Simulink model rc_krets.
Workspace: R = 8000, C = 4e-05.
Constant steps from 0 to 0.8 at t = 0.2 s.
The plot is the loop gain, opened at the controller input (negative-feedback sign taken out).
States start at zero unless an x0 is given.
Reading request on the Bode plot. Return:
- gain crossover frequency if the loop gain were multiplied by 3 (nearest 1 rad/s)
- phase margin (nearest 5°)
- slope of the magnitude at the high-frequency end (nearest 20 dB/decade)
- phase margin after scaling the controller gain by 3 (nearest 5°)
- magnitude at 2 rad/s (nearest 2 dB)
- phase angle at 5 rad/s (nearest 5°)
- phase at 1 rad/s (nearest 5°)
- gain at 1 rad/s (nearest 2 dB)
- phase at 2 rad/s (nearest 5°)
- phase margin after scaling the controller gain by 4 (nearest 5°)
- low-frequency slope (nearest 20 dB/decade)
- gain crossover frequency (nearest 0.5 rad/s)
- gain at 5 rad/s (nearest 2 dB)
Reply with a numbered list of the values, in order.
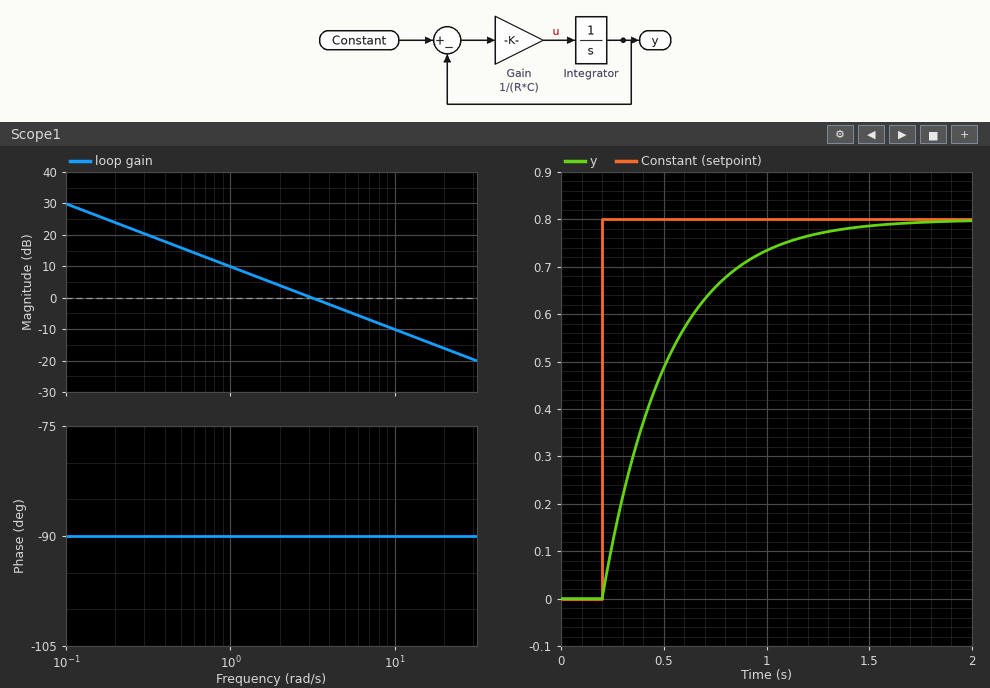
1. 9 rad/s
2. 90°
3. -20 dB/decade
4. 90°
5. 4 dB
6. -90°
7. -90°
8. 10 dB
9. -90°
10. 90°
11. -20 dB/decade
12. 3.0 rad/s
13. -4 dB
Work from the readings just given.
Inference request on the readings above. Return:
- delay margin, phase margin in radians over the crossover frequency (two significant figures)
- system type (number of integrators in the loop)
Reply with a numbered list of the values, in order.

1. 0.52 s
2. 1
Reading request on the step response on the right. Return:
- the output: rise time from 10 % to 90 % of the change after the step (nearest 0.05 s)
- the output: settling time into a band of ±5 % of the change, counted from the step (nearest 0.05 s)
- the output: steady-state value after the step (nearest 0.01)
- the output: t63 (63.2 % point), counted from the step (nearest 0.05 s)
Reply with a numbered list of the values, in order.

1. 0.70 s
2. 0.95 s
3. 0.80
4. 0.30 s
